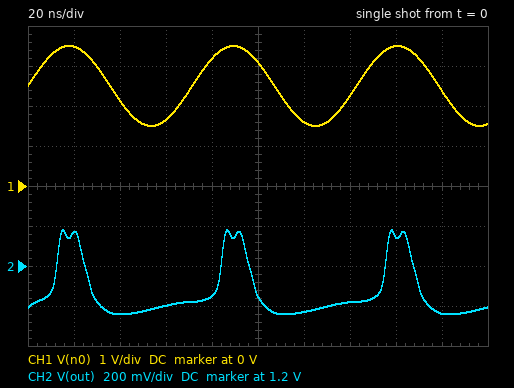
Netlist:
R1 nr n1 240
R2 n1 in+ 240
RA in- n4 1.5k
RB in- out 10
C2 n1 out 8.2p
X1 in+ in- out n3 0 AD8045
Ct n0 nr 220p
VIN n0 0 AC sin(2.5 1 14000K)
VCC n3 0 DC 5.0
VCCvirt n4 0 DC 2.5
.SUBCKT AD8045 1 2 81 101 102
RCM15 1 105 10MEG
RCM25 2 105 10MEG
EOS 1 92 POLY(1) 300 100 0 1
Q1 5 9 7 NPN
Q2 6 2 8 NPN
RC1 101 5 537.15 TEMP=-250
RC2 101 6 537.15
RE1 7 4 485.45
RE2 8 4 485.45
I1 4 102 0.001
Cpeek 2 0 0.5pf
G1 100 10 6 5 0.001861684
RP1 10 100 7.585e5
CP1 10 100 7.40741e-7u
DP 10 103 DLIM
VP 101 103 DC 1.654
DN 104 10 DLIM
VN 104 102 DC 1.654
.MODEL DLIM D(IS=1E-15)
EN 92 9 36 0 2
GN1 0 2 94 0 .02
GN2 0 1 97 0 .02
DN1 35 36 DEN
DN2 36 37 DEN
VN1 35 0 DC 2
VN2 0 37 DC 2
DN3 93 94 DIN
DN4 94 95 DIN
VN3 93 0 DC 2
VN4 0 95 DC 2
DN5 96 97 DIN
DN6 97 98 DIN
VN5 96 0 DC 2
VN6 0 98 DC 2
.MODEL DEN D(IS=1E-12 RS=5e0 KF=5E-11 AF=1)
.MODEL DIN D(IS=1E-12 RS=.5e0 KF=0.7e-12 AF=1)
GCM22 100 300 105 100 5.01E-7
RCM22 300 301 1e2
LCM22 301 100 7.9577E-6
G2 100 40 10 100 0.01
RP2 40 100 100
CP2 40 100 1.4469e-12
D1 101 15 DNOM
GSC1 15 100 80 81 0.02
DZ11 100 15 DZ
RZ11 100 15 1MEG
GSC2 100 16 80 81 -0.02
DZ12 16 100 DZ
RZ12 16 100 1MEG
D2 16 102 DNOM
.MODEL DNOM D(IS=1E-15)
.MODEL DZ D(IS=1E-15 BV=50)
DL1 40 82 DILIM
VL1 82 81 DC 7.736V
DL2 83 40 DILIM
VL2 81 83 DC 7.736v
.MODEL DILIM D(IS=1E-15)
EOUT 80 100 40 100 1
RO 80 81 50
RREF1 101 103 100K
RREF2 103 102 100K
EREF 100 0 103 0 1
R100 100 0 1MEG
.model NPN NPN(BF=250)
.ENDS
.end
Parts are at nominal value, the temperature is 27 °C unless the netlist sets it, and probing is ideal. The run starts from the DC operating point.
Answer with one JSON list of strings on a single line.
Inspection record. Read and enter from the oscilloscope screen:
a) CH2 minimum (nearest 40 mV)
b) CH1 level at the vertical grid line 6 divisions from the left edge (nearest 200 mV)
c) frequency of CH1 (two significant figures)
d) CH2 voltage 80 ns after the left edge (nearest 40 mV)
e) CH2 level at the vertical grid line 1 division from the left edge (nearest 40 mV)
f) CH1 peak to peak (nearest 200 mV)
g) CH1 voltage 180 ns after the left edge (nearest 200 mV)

["960 mV", "1.6 V", "14 MHz", "1.04 V", "1.36 V", "2.0 V", "2.4 V"]
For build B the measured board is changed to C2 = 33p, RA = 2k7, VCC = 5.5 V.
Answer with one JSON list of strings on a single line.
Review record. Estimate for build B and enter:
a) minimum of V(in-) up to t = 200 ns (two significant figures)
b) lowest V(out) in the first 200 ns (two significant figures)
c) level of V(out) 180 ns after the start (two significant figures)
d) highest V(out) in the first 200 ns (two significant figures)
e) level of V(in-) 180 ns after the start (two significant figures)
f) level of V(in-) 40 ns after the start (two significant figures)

["880 mV", "870 mV", "900 mV", "1.3 V", "910 mV", "890 mV"]
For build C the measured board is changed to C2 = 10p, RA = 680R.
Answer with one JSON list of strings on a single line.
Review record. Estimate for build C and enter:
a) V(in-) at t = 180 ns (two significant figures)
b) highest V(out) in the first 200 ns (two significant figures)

["1.0 V", "1.5 V"]
